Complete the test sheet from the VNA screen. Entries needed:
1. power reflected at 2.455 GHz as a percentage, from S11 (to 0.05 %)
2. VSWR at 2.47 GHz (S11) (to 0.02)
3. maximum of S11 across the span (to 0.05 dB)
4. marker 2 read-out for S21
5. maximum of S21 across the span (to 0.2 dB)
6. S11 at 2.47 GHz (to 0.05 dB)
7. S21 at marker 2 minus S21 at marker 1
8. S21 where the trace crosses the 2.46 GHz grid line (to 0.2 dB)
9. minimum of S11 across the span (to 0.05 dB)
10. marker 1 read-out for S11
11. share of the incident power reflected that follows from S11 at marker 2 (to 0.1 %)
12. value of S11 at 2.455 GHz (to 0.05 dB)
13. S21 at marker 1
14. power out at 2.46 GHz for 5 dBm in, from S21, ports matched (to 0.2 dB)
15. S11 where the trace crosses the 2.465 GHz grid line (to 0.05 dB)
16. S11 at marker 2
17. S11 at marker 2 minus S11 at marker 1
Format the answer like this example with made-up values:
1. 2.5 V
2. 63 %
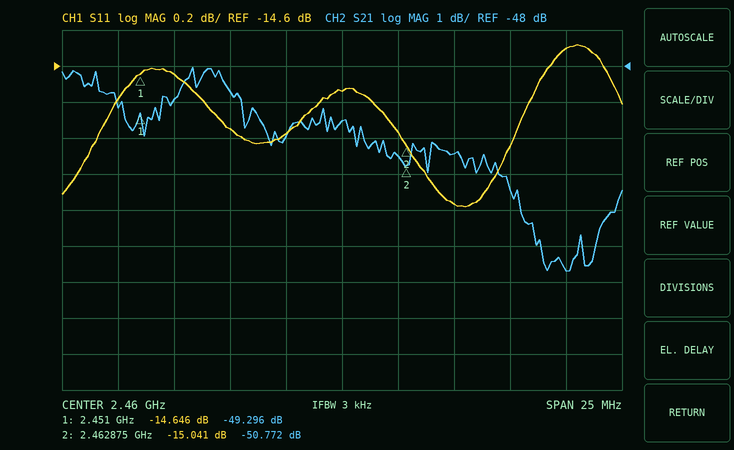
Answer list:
1. 3.20 %
2. 1.46
3. -14.50 dB
4. -50.772 dB
5. -48.0 dB
6. -14.50 dB
7. -1.476 dB
8. -49.6 dB
9. -15.40 dB
10. -14.646 dB
11. 3.1 %
12. -14.95 dB
13. -49.296 dB
14. -44.6 dBm
15. -15.35 dB
16. -15.041 dB
17. -0.395 dB
